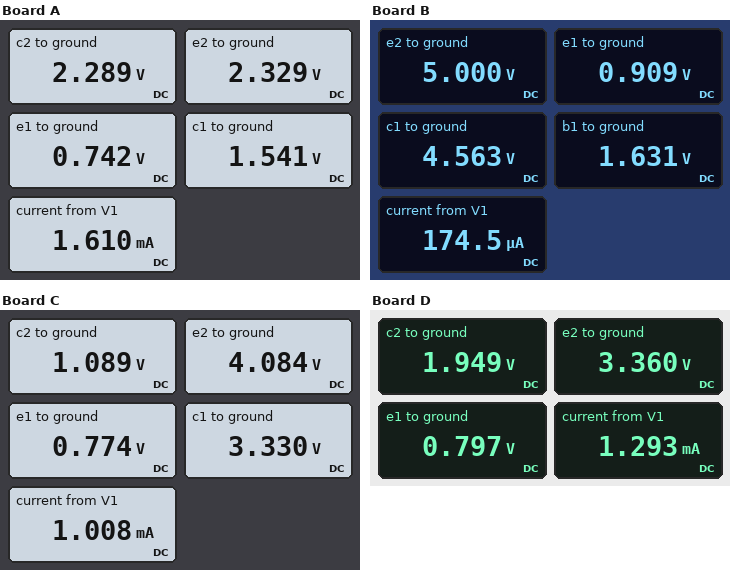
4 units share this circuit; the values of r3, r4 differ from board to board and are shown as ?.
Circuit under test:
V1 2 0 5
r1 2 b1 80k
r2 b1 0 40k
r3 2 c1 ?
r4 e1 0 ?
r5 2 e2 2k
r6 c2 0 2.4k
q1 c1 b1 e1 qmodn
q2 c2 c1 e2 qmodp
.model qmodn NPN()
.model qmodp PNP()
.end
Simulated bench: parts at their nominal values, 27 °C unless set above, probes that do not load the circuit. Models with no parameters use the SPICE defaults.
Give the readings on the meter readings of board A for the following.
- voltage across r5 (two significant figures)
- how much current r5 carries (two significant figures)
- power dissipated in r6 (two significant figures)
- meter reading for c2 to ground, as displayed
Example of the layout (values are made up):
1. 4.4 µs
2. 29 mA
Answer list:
1. 2.7 V
2. 1.3 mA
3. 2.2 mW
4. 2.289 V
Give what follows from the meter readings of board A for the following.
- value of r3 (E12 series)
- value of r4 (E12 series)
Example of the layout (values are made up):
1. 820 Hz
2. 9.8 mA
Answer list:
1. 15 kΩ
2. 1.2 kΩ
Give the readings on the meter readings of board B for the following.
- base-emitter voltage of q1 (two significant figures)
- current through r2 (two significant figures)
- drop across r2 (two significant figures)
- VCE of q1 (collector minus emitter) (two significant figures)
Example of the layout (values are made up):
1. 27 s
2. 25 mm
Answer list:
1. 720 mV
2. 41 µA
3. 1.6 V
4. 3.7 V
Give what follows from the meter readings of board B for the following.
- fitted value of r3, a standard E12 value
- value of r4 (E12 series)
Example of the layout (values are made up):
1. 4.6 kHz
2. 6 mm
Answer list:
1. 3.3 kΩ
2. 6.8 kΩ
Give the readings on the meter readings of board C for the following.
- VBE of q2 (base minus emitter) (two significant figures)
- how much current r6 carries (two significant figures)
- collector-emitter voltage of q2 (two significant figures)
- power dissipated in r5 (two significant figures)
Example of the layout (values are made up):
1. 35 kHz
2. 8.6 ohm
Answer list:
1. -750 mV
2. 450 µA
3. -3.0 V
4. 420 µW
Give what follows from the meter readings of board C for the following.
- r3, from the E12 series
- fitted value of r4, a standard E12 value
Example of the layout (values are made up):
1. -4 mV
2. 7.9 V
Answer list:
1. 3.3 kΩ
2. 1.5 kΩ
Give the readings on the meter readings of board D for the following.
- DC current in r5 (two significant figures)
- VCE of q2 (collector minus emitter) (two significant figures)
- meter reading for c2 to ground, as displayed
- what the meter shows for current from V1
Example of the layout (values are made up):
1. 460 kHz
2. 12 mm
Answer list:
1. 820 µA
2. -1.4 V
3. 1.949 V
4. 1.293 mA
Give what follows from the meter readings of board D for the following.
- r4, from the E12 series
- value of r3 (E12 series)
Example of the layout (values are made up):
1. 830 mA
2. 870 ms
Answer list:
1. 1.8 kΩ
2. 5.6 kΩ
